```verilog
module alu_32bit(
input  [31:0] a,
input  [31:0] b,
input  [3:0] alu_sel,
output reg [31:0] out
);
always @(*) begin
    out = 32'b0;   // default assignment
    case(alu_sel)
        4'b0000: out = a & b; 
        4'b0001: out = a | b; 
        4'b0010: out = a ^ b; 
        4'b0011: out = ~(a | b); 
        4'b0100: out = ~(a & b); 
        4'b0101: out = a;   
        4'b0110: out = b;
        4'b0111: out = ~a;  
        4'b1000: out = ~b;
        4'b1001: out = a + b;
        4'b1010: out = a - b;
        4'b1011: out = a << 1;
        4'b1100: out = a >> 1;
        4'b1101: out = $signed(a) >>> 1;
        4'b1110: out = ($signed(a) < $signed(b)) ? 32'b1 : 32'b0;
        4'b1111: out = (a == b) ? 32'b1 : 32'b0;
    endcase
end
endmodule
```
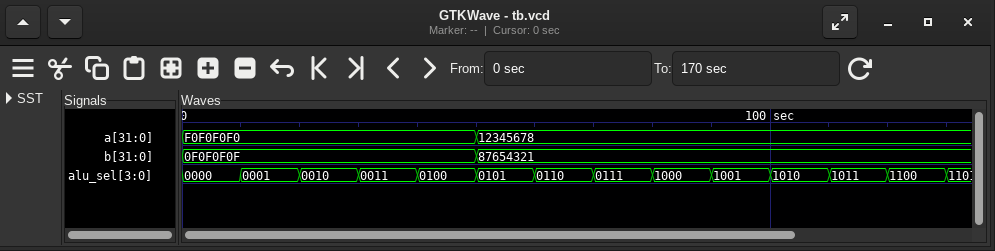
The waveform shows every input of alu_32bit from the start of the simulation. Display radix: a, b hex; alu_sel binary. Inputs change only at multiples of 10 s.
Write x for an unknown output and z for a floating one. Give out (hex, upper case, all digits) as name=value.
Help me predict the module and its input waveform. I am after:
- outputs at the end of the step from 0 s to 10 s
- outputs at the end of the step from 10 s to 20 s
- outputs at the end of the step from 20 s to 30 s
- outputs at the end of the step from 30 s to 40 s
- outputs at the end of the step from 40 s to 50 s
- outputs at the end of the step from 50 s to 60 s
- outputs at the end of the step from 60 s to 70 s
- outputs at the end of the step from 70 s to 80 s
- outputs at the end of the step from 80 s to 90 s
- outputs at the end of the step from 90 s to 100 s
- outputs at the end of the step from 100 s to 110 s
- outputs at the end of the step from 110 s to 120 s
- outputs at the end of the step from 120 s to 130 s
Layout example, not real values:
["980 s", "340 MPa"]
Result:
["out=00000000", "out=FFFFFFFF", "out=FFFFFFFF", "out=00000000", "out=FFFFFFFF", "out=12345678", "out=87654321", "out=EDCBA987", "out=789ABCDE", "out=99999999", "out=8ACF1357", "out=2468ACF0", "out=091A2B3C"]
